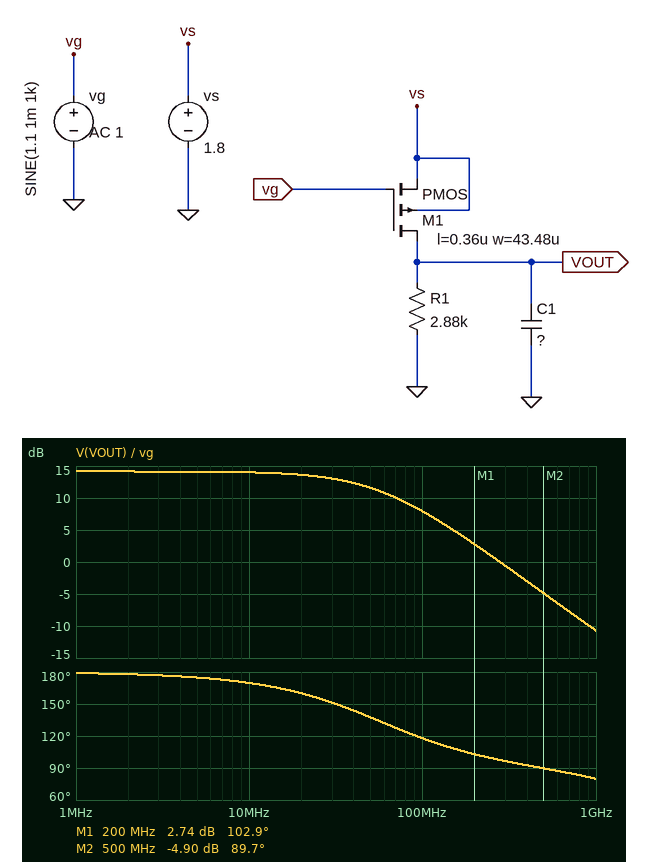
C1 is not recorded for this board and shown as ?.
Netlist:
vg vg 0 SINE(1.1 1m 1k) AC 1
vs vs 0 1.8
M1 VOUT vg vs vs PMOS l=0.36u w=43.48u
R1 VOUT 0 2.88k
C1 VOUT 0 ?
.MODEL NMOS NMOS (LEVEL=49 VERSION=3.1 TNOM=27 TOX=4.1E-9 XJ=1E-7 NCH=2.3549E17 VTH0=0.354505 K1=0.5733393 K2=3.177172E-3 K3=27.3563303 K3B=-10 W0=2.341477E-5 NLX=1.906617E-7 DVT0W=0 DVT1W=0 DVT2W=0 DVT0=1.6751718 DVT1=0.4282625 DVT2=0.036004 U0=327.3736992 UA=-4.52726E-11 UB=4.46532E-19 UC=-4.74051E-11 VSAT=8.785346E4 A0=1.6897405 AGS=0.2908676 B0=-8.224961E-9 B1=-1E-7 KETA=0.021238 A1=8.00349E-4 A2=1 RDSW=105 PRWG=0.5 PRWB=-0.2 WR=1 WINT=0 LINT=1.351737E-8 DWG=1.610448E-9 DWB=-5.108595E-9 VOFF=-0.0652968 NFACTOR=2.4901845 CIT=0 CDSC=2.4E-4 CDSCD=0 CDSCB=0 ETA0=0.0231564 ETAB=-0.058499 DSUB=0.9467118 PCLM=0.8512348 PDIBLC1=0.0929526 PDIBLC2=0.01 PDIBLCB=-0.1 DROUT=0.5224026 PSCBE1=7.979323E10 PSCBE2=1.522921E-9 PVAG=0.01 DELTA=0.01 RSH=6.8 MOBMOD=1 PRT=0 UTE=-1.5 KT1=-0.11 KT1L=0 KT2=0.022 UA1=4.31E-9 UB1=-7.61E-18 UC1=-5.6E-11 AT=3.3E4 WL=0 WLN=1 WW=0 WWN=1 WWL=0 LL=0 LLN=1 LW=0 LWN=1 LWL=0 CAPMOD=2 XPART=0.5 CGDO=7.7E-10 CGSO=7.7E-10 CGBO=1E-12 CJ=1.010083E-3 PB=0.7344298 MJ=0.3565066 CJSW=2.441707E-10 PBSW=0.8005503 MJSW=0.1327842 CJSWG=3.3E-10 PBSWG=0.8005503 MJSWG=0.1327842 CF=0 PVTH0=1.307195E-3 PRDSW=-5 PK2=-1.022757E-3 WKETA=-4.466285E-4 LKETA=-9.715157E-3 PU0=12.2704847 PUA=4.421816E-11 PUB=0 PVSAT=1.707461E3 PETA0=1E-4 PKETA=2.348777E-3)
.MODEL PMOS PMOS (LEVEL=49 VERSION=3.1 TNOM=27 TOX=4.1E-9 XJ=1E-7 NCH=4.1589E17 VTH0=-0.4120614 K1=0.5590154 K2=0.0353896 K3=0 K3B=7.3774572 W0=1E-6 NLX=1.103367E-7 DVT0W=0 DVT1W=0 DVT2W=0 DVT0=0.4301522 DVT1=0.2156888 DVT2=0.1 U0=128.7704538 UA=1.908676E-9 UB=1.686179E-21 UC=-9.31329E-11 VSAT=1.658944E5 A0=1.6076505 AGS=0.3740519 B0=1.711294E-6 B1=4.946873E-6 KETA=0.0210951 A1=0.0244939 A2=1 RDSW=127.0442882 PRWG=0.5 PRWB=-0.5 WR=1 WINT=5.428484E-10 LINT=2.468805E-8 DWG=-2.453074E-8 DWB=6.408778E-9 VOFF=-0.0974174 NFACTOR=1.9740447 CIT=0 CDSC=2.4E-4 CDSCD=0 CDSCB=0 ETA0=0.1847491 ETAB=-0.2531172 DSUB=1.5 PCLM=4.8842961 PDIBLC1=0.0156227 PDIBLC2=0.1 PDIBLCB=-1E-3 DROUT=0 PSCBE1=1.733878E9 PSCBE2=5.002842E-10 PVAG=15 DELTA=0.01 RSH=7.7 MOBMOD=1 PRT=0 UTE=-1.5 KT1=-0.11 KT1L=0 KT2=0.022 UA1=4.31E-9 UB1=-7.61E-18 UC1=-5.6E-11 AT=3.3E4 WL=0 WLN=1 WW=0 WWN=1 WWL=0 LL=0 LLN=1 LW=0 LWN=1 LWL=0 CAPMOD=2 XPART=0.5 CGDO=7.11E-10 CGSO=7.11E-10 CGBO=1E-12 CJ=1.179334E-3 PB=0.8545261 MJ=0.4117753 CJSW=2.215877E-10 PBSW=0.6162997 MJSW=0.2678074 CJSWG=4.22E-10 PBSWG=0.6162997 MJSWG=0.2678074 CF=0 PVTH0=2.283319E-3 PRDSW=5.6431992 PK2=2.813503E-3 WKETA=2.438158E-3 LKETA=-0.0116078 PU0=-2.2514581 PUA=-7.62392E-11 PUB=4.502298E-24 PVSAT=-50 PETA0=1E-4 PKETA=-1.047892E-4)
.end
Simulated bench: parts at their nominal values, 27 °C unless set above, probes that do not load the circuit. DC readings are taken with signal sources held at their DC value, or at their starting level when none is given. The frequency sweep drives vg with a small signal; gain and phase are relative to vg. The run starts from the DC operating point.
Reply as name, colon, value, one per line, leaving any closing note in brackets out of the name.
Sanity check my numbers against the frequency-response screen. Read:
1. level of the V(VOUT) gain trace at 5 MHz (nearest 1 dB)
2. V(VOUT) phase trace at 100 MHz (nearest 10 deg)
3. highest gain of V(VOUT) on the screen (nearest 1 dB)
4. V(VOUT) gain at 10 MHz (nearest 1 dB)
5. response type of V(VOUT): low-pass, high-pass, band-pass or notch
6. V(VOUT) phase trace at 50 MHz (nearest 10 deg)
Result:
level of the V(VOUT) gain trace at 5 MHz: 14 dB
V(VOUT) phase trace at 100 MHz: 120 deg
highest gain of V(VOUT) on the screen: 14 dB
V(VOUT) gain at 10 MHz: 14 dB
response type of V(VOUT): low-pass, high-pass, band-pass or notch: low-pass
V(VOUT) phase trace at 50 MHz: 140 deg
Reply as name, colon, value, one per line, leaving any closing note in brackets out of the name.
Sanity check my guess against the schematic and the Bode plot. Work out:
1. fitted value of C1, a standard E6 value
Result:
fitted value of C1, a standard E6 value: 1 pF
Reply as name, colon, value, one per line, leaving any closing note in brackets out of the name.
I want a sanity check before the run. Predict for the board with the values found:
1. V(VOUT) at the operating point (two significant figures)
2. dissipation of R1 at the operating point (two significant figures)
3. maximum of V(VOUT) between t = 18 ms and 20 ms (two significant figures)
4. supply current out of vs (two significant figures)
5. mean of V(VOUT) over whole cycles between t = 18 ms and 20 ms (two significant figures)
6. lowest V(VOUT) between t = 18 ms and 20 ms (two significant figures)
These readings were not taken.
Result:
V(VOUT) at the operating point: 670 mV
dissipation of R1 at the operating point: 150 µW
maximum of V(VOUT) between t = 18 ms and 20 ms: 670 mV
supply current out of vs: 230 µA
mean of V(VOUT) over whole cycles between t = 18 ms and 20 ms: 670 mV
lowest V(VOUT) between t = 18 ms and 20 ms: 660 mV
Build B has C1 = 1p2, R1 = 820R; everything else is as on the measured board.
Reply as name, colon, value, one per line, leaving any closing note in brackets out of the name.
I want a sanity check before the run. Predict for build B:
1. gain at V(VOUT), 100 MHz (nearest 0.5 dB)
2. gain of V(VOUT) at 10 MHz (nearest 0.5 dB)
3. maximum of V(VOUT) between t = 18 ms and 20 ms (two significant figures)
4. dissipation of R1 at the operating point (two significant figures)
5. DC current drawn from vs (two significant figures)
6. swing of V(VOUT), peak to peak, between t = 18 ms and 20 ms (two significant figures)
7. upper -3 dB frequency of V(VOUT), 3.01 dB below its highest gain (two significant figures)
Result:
gain at V(VOUT), 100 MHz: 2.5 dB
gain of V(VOUT) at 10 MHz: 4.0 dB
maximum of V(VOUT) between t = 18 ms and 20 ms: 200 mV
dissipation of R1 at the operating point: 47 µW
DC current drawn from vs: 240 µA
swing of V(VOUT), peak to peak, between t = 18 ms and 20 ms: 3.1 mV
upper -3 dB frequency of V(VOUT), 3.01 dB below its highest gain: 160 MHz
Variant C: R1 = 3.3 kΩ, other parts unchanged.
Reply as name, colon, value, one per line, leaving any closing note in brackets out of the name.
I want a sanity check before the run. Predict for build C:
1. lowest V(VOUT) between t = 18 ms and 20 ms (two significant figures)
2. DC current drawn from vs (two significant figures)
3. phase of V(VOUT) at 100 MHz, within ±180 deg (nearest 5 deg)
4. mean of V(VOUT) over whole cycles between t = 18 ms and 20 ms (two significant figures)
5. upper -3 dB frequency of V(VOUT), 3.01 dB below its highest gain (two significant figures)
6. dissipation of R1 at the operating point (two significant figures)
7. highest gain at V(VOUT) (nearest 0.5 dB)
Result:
lowest V(VOUT) between t = 18 ms and 20 ms: 750 mV
DC current drawn from vs: 230 µA
phase of V(VOUT) at 100 MHz, within ±180 deg: 115 deg
mean of V(VOUT) over whole cycles between t = 18 ms and 20 ms: 760 mV
upper -3 dB frequency of V(VOUT), 3.01 dB below its highest gain: 49 MHz
dissipation of R1 at the operating point: 170 µW
highest gain at V(VOUT): 15.0 dB
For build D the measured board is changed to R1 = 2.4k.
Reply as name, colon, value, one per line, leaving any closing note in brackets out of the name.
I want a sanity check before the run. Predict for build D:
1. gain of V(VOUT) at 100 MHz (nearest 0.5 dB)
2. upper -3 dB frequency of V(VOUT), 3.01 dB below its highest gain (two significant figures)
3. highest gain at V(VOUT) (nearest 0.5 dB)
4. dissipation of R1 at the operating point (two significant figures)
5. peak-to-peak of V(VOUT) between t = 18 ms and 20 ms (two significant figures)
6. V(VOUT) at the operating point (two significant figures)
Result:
gain of V(VOUT) at 100 MHz: 7.5 dB
upper -3 dB frequency of V(VOUT), 3.01 dB below its highest gain: 66 MHz
highest gain at V(VOUT): 12.5 dB
dissipation of R1 at the operating point: 130 µW
peak-to-peak of V(VOUT) between t = 18 ms and 20 ms: 8.6 mV
V(VOUT) at the operating point: 560 mV
